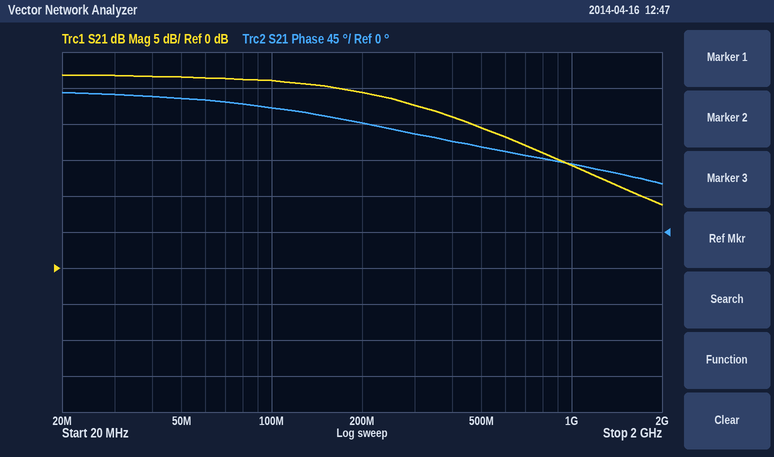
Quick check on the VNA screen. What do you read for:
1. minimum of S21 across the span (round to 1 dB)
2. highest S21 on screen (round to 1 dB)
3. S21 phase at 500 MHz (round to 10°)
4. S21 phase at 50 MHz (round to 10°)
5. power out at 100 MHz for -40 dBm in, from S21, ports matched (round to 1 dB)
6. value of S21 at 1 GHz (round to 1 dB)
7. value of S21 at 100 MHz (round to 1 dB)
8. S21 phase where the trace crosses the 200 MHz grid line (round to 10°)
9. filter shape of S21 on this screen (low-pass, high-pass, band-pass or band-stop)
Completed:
9 dB
27 dB
110°
170°
-14 dBm
14 dB
26 dB
140°
low-pass
